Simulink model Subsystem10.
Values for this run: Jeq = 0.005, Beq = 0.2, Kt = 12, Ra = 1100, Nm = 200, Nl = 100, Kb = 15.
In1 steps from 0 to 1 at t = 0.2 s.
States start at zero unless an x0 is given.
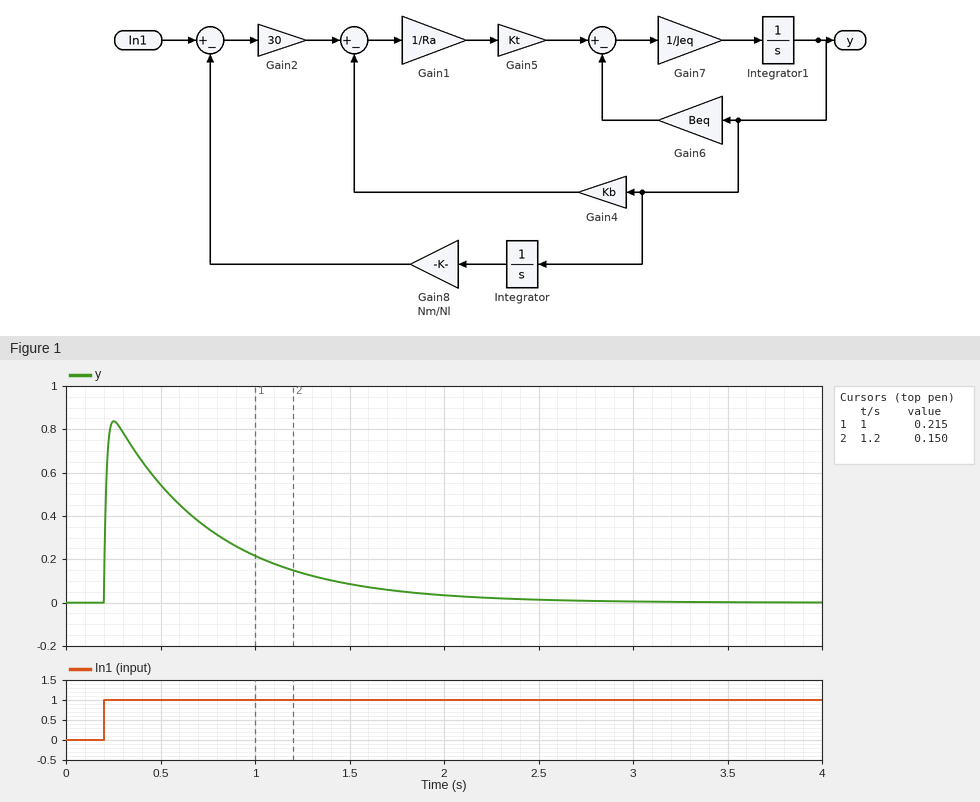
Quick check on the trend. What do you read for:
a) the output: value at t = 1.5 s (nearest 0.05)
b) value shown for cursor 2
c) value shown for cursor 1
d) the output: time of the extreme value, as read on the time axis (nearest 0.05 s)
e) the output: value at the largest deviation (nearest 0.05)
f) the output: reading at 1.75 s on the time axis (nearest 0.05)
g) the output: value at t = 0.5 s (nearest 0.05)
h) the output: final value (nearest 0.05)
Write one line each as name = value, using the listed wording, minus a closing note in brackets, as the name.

the output: value at t = 1.5 s = 0.10
value shown for cursor 2 = 0.150
value shown for cursor 1 = 0.215
the output: time of the extreme value, as read on the time axis = 0.25 s
the output: value at the largest deviation = 0.85
the output: reading at 1.75 s on the time axis = 0.05
the output: value at t = 0.5 s = 0.55
the output: final value = 0.00
